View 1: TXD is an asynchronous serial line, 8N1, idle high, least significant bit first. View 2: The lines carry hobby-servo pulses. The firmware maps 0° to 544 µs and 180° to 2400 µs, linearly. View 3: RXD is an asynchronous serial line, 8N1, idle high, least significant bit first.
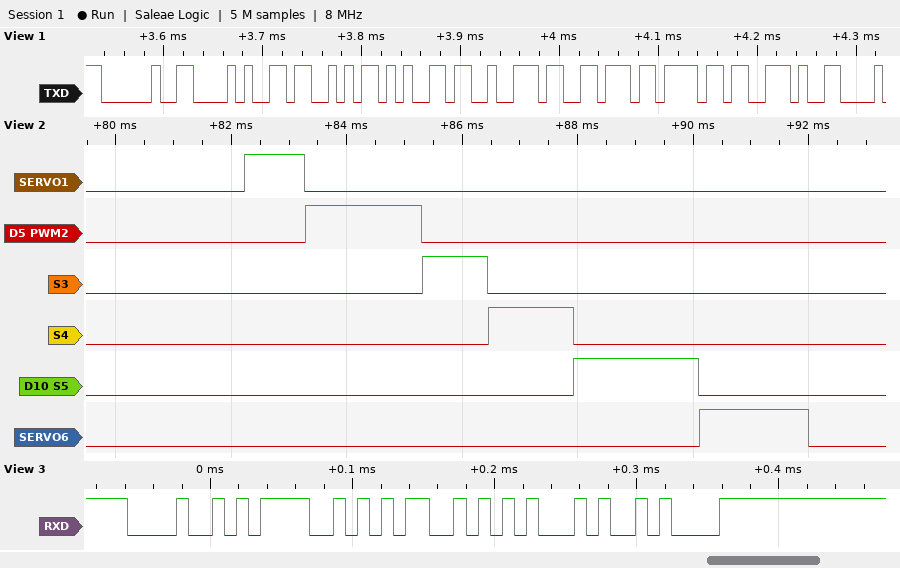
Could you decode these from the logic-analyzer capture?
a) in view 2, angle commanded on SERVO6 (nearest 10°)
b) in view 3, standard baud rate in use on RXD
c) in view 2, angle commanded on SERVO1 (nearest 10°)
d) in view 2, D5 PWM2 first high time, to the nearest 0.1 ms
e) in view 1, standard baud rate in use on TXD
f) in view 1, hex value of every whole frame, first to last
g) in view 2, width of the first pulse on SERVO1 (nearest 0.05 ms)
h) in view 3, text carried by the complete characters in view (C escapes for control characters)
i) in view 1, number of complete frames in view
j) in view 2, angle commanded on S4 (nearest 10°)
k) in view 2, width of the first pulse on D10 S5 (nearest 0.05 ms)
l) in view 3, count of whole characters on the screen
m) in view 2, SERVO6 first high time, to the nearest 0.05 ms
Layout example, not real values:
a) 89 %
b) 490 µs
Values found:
a) 130°
b) 115200 baud
c) 50°
d) 2.0 ms
e) 115200 baud
f) 20 28 53 65 72 76 6F 2E
g) 1.05 ms
h) "HOME\n"
i) 8
j) 90°
k) 2.15 ms
l) 5
m) 1.90 ms
